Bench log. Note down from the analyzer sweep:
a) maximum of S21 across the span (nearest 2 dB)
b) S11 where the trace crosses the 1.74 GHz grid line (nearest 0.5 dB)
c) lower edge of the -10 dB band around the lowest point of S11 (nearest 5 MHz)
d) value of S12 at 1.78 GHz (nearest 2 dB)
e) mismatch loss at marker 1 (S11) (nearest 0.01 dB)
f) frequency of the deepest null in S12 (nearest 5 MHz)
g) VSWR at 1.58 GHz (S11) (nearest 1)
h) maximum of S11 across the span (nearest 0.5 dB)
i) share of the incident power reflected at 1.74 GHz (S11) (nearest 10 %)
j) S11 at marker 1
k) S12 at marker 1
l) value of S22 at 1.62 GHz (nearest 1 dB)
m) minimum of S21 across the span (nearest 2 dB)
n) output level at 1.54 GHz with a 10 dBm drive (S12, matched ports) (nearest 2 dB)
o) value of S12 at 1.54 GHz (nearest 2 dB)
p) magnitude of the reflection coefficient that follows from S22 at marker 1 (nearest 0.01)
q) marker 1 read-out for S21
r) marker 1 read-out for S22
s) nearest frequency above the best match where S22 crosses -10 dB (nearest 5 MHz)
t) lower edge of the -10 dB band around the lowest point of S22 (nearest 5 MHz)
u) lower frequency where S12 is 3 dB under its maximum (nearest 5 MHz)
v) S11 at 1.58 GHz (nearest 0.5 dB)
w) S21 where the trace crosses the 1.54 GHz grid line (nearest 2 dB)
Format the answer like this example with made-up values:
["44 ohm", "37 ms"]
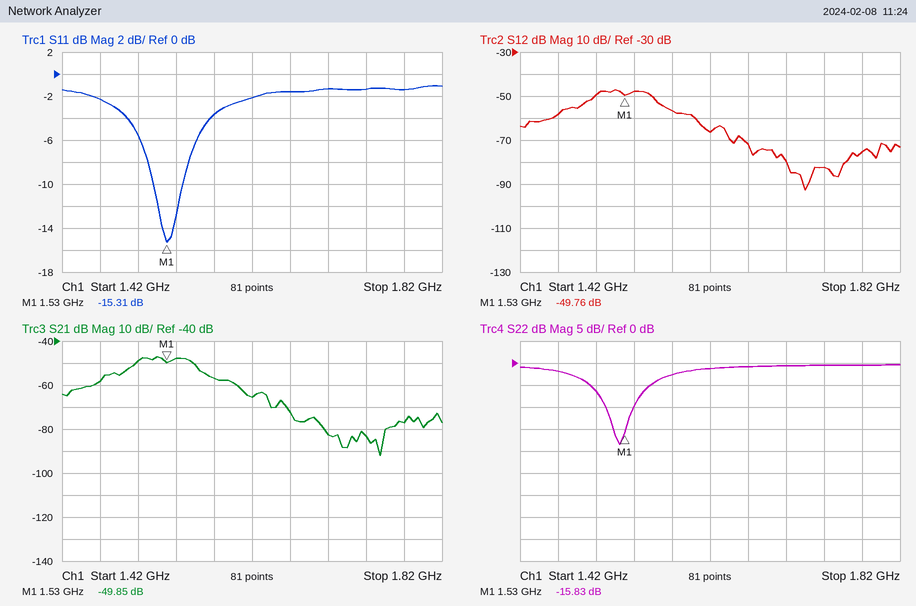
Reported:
["-48 dB", "-1.5 dB", "1.515 GHz", "-76 dB", "0.13 dB", "1.720 GHz", "5", "-1.0 dB", "70 %", "-15.31 dB", "-49.76 dB", "-1 dB", "-92 dB", "-38 dBm", "-48 dB", "0.16", "-49.85 dB", "-15.83 dB", "1.540 GHz", "1.510 GHz", "1.500 GHz", "-3.5 dB", "-48 dB"]
